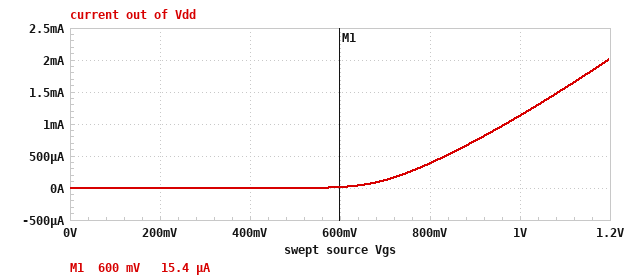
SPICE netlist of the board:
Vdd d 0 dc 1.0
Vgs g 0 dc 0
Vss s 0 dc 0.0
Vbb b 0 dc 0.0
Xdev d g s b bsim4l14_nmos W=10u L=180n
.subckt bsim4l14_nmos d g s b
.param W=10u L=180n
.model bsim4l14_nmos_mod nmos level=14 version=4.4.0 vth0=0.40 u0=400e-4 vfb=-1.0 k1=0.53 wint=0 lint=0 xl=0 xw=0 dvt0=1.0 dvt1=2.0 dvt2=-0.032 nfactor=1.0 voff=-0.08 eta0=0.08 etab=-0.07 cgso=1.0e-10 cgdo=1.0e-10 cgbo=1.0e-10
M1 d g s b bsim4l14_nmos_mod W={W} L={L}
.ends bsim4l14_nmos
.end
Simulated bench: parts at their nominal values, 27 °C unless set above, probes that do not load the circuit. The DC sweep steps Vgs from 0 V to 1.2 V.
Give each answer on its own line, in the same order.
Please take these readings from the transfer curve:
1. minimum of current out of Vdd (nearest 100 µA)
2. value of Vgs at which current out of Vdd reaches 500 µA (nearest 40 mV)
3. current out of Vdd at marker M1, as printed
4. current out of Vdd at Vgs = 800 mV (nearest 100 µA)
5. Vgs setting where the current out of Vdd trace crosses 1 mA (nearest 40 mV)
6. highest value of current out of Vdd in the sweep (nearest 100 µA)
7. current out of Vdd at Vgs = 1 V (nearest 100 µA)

0 A
840 mV
15.4 µA
400 µA
960 mV
2.0 mA
1.1 mA
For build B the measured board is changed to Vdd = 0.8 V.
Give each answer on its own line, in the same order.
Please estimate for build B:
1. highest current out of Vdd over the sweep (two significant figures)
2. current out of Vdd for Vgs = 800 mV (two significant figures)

1.9 mA
360 µA
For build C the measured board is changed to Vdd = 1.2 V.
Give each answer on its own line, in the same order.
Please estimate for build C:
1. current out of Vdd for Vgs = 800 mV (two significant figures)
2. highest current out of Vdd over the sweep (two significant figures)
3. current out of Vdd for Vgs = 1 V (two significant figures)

410 µA
2.1 mA
1.2 mA
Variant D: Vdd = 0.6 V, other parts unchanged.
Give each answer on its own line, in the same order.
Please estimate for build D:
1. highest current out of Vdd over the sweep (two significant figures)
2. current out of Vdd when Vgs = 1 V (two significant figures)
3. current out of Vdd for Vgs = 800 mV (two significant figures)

1.8 mA
1.0 mA
340 µA
